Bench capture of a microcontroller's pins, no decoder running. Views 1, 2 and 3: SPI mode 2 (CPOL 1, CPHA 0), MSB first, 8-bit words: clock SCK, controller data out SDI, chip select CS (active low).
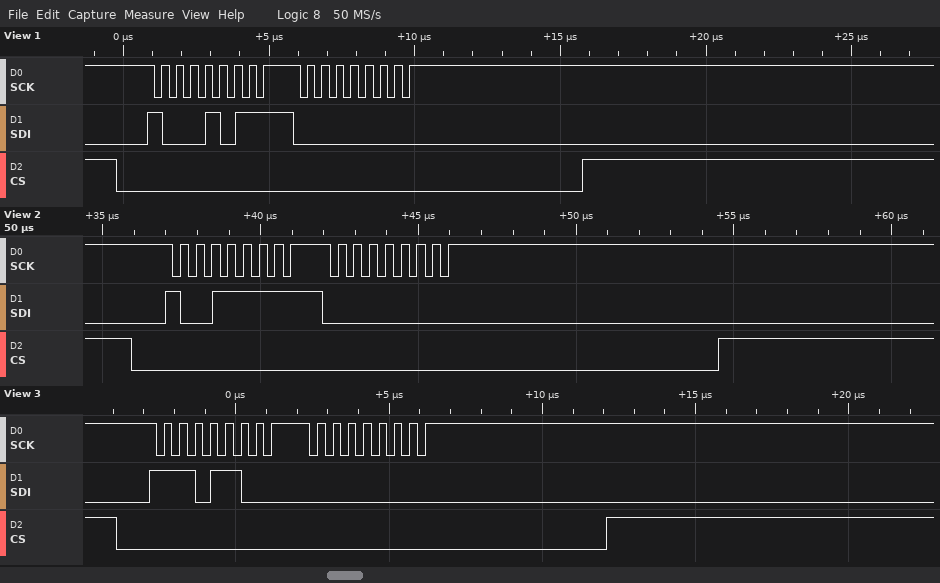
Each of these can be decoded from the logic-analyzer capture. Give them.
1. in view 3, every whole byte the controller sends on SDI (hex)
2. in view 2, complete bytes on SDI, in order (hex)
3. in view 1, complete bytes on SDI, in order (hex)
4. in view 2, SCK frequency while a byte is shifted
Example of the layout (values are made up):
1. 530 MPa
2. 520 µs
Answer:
1. EC 00
2. 9F 00
3. 0x8B 0x00
4. 2 MHz
